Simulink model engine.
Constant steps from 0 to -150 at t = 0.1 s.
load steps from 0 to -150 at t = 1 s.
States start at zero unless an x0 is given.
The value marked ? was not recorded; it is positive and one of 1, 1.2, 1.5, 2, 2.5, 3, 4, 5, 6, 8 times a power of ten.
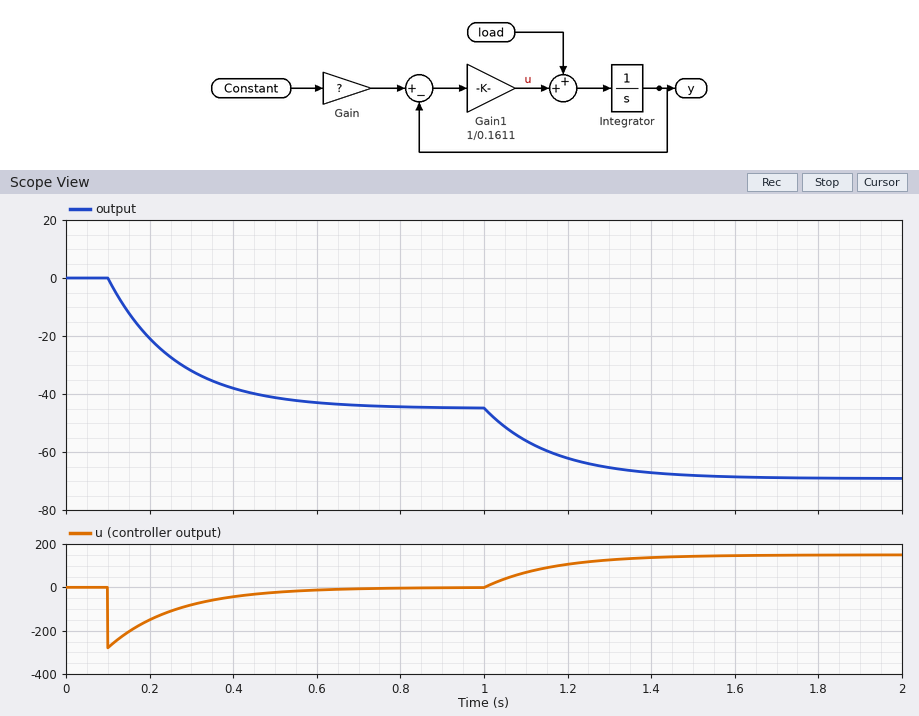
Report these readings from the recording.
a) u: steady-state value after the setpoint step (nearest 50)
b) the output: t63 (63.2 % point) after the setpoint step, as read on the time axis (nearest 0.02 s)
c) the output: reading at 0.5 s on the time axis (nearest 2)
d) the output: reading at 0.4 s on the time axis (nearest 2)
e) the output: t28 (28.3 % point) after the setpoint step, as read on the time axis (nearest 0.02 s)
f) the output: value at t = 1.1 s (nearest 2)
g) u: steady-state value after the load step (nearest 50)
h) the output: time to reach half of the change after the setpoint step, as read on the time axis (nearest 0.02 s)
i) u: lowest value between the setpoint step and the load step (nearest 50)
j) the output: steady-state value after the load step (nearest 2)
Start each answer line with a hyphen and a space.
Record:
- 0
- 0.26 s
- -42
- -38
- 0.16 s
- -56
- 150
- 0.22 s
- -300
- -70
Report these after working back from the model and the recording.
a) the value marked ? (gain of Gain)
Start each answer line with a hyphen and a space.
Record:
- 0.3
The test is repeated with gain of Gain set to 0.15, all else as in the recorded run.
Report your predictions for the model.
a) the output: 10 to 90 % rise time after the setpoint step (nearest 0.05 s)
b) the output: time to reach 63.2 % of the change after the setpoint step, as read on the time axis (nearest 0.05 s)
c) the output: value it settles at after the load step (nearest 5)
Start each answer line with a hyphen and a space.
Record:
- 0.35 s
- 0.25 s
- -45
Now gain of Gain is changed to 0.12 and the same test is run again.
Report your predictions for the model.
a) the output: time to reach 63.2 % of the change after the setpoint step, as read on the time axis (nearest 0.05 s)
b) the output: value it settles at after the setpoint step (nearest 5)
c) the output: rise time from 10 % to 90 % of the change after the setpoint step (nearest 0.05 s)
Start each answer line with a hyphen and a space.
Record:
- 0.25 s
- -20
- 0.35 s
